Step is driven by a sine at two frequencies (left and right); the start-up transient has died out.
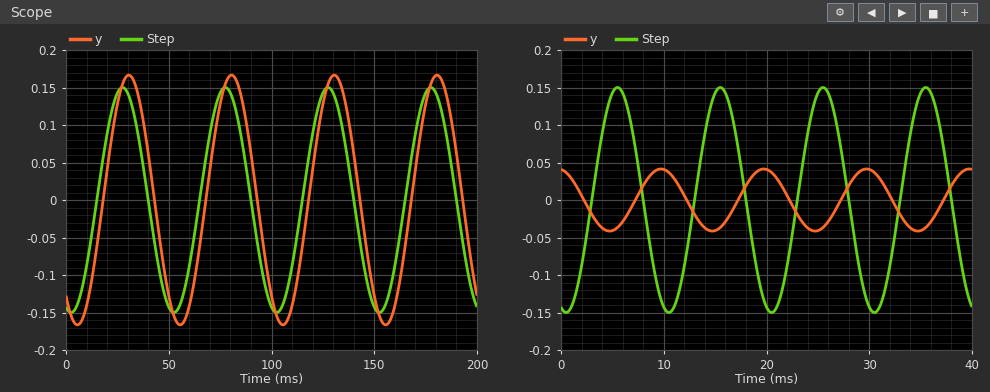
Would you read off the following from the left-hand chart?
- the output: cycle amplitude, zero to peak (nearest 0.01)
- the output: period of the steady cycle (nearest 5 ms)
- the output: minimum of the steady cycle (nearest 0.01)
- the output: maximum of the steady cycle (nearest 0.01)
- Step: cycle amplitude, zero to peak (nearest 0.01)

0.17
50 ms
-0.17
0.17
0.15
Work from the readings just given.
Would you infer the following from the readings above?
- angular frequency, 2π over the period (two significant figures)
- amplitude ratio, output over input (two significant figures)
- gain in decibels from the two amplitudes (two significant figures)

0.13 rad/ms
1.1
1.1 dB
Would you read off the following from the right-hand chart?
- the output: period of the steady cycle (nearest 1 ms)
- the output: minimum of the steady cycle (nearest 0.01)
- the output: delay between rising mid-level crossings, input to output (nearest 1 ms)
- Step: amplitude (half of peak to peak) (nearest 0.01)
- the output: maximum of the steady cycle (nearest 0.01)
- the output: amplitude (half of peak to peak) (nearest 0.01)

10 ms
-0.04
4 ms
0.15
0.04
0.04
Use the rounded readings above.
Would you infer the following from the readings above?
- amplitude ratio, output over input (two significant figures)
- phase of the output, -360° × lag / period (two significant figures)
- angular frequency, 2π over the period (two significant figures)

0.27
-140°
0.63 rad/ms
